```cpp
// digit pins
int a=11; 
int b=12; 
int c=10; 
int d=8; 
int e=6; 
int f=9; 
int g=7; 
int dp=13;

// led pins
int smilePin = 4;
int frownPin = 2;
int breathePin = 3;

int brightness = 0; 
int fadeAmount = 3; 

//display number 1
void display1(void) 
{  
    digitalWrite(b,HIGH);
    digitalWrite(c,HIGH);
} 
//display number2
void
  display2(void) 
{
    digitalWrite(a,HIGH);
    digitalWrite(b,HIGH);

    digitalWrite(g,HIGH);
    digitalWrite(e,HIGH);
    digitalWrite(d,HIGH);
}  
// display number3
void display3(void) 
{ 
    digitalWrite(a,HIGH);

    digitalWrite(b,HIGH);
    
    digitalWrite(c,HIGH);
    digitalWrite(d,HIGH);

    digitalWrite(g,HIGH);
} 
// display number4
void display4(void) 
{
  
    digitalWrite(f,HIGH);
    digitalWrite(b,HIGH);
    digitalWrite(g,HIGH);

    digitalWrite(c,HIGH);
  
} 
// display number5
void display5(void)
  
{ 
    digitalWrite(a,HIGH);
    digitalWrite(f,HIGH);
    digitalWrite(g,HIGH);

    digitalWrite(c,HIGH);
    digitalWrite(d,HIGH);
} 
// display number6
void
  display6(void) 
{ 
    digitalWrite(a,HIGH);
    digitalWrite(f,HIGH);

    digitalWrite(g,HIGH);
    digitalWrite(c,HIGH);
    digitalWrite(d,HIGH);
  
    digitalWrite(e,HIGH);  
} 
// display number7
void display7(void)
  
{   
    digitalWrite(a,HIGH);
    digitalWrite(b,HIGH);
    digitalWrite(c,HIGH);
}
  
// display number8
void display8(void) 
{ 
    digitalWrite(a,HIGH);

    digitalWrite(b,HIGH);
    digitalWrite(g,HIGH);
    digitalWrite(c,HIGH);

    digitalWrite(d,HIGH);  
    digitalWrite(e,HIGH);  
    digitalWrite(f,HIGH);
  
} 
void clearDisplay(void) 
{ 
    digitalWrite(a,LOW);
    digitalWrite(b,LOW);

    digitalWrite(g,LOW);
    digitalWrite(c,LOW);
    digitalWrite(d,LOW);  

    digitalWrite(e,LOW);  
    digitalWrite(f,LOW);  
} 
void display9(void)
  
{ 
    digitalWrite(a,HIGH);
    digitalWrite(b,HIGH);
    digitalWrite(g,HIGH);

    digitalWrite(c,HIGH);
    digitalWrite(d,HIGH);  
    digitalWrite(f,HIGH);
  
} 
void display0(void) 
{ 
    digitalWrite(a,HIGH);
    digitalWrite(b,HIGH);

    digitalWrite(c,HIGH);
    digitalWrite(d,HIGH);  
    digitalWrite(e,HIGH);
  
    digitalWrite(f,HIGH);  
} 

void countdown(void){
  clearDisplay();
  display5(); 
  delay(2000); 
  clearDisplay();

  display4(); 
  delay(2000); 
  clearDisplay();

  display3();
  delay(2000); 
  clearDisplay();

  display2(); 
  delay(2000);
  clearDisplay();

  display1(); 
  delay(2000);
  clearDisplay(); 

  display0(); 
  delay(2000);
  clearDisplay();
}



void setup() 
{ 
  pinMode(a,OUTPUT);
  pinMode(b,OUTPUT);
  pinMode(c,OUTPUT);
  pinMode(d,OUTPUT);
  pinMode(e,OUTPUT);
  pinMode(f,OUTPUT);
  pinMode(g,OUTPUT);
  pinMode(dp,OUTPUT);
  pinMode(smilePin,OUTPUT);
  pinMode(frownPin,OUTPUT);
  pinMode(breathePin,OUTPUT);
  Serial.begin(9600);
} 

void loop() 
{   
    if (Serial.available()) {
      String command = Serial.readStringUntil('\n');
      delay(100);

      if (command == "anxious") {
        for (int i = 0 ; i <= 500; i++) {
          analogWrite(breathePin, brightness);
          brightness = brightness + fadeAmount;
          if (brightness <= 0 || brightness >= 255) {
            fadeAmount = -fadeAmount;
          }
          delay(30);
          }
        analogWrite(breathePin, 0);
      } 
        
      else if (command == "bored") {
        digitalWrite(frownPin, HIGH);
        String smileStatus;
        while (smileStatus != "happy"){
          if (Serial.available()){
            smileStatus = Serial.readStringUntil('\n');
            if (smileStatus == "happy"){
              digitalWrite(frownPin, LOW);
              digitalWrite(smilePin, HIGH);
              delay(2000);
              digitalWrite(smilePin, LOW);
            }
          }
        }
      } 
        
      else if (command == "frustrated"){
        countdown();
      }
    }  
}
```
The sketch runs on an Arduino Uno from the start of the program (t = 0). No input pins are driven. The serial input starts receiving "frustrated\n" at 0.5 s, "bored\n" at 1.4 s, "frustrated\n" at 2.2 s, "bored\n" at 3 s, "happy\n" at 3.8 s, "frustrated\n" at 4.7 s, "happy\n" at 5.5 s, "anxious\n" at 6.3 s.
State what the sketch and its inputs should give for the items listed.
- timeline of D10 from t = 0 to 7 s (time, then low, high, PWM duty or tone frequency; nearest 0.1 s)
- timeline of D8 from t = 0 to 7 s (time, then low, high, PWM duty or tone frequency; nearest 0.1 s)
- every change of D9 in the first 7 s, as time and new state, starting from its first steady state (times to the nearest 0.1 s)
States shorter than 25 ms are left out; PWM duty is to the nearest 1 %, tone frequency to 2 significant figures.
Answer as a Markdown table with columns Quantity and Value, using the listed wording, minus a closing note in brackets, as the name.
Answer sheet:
| Quantity | Value |
|---|---|
| timeline of D10 from t = 0 to 7 s | 0 s low; 0.6 s high; 6.6 s low |
| timeline of D8 from t = 0 to 7 s | 0 s low; 0.6 s high; 2.6 s low; 4.6 s high |
| every change of D9 in the first 7 s, as time and new state, starting from its first steady state | 0 s low; 0.6 s high; 4.6 s low |
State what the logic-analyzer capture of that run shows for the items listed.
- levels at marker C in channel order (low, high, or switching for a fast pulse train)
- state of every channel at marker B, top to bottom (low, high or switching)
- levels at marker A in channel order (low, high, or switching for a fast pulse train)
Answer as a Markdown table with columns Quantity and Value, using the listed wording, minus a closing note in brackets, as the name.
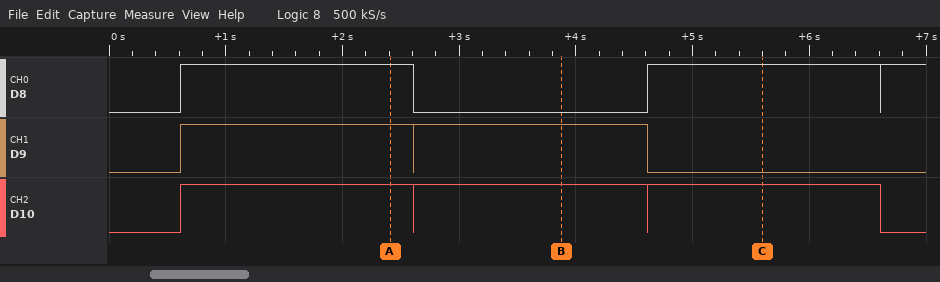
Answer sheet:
| Quantity | Value |
|---|---|
| levels at marker C in channel order | D8 high, D9 low, D10 high |
| state of every channel at marker B, top to bottom | D8 low, D9 high, D10 high |
| levels at marker A in channel order | D8 high, D9 high, D10 high |
